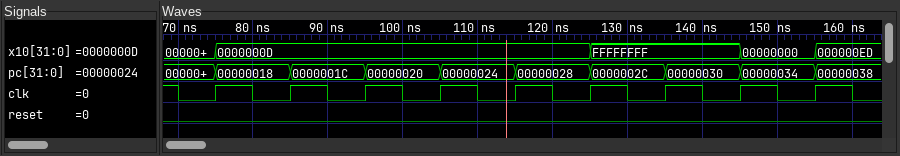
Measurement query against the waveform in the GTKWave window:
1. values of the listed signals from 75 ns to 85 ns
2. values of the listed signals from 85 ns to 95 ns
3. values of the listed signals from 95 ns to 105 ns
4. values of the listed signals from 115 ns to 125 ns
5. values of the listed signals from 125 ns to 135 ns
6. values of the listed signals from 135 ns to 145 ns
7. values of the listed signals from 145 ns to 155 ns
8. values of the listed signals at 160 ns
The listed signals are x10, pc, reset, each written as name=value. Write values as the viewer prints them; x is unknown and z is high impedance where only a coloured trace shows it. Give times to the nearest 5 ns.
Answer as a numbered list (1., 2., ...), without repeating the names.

1. x10=0000000D, pc=00000018, reset=0
2. x10=0000000D, pc=0000001C, reset=0
3. x10=0000000D, pc=00000020, reset=0
4. x10=0000000D, pc=00000028, reset=0
5. x10=FFFFFFFF, pc=0000002C, reset=0
6. x10=FFFFFFFF, pc=00000030, reset=0
7. x10=00000000, pc=00000034, reset=0
8. x10=000000ED, pc=00000038, reset=0
